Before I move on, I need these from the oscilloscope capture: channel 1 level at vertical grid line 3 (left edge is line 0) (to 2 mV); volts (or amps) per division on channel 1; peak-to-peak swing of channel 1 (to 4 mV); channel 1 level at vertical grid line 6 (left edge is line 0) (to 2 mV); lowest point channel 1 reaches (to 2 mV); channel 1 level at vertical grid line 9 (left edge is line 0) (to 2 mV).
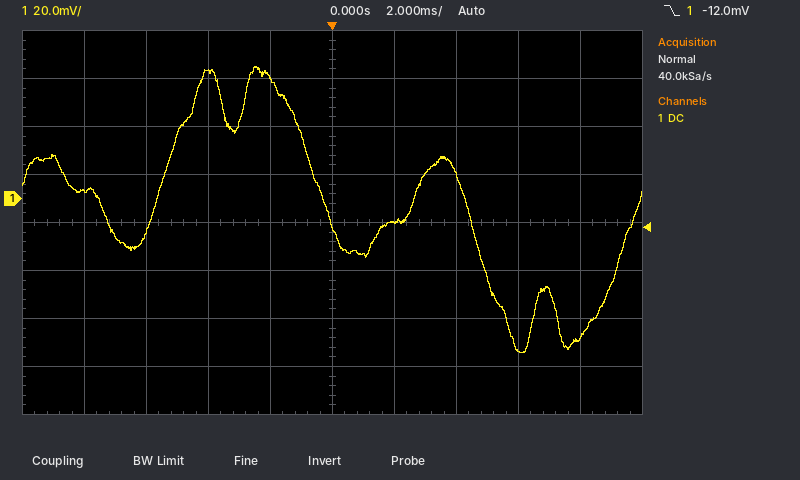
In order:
52 mV
20 mV
120 mV
-10 mV
-64 mV
-58 mV
